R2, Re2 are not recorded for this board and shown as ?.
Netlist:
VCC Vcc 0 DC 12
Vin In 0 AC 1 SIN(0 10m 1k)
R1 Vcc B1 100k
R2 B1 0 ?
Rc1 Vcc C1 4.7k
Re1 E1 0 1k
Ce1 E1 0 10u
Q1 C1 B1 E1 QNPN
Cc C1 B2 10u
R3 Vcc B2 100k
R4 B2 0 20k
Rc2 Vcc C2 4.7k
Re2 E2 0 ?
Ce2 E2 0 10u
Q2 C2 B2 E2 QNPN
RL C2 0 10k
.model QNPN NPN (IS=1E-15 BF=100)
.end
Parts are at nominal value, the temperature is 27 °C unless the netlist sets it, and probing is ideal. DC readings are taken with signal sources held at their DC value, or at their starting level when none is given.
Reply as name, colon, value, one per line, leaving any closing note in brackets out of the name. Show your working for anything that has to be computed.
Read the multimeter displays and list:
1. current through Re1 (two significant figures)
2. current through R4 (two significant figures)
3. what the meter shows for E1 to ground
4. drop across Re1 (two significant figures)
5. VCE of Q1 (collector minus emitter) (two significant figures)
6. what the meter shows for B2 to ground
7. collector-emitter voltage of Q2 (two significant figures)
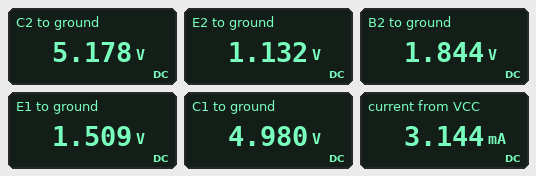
current through Re1: (1.509 V) / 1 kΩ = 1.5 mA
current through R4: (1.844 V) / 20 kΩ = 92 µA
what the meter shows for E1 to ground: 1.509 V
drop across Re1: 1.509 V = 1.5 V
VCE of Q1 (collector minus emitter): 4.98 V - 1.509 V = 3.5 V
what the meter shows for B2 to ground: 1.844 V
collector-emitter voltage of Q2: 5.178 V - 1.132 V = 4.0 V
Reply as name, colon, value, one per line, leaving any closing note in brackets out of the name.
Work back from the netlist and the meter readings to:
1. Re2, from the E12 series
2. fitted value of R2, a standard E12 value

Re2, from the E12 series: 1.2 kΩ
fitted value of R2, a standard E12 value: 27 kΩ
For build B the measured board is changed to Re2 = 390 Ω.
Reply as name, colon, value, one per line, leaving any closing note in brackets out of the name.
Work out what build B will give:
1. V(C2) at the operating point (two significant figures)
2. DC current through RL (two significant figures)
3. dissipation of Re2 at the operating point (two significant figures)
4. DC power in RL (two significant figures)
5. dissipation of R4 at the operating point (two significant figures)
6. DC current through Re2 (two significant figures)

V(C2) at the operating point: 1.1 V
DC current through RL: 110 µA
dissipation of Re2 at the operating point: 2.0 mW
DC power in RL: 110 µW
dissipation of R4 at the operating point: 130 µW
DC current through Re2: 2.2 mA
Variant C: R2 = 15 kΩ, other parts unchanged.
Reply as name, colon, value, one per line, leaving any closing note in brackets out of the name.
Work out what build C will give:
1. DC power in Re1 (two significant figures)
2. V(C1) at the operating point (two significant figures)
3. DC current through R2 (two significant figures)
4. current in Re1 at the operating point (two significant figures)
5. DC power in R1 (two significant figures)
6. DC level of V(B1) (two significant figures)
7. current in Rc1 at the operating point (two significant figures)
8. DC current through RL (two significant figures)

DC power in Re1: 580 µW
V(C1) at the operating point: 8.5 V
DC current through R2: 98 µA
current in Re1 at the operating point: 760 µA
DC power in R1: 1.1 mW
DC level of V(B1): 1.5 V
current in Rc1 at the operating point: 750 µA
DC current through RL: 520 µA
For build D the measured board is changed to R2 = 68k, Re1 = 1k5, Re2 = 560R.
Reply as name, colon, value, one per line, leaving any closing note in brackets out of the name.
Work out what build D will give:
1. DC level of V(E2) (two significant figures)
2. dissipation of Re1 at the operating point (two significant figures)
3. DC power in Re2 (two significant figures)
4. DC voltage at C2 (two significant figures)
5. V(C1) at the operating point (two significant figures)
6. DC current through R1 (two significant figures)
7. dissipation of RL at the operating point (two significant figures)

DC level of V(E2): 980 mV
dissipation of Re1 at the operating point: 5.6 mW
DC power in Re2: 1.7 mW
DC voltage at C2: 2.6 V
V(C1) at the operating point: 3.0 V
DC current through R1: 84 µA
dissipation of RL at the operating point: 680 µW
